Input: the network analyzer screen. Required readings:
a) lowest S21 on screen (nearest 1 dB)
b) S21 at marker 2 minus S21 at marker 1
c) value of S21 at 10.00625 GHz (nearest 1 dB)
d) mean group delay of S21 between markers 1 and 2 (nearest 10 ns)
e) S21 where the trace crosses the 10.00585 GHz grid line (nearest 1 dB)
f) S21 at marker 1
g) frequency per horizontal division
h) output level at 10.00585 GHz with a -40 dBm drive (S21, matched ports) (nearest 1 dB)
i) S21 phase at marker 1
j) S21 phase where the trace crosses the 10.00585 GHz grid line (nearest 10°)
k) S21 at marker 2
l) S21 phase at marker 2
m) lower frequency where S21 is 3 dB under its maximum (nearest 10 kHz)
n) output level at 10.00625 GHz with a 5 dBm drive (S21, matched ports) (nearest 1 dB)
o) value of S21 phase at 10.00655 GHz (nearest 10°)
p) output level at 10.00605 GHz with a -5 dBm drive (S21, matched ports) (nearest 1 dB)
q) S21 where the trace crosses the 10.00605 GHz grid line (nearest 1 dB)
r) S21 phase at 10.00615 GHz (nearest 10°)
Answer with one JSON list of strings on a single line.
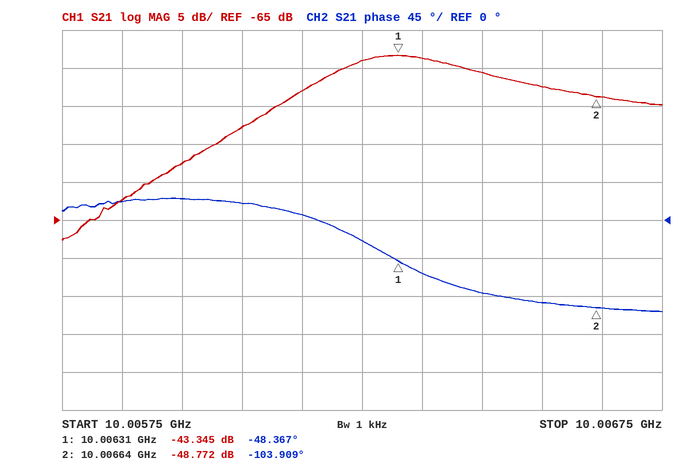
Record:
["-68 dB", "-5.427 dB", "-44 dB", "470 ns", "-62 dB", "-43.345 dB", "100 kHz", "-102 dBm", "-48.367°", "20°", "-48.772 dB", "-103.909°", "10.00619 GHz", "-39 dBm", "-100°", "-58 dBm", "-53 dB", "10°"]
